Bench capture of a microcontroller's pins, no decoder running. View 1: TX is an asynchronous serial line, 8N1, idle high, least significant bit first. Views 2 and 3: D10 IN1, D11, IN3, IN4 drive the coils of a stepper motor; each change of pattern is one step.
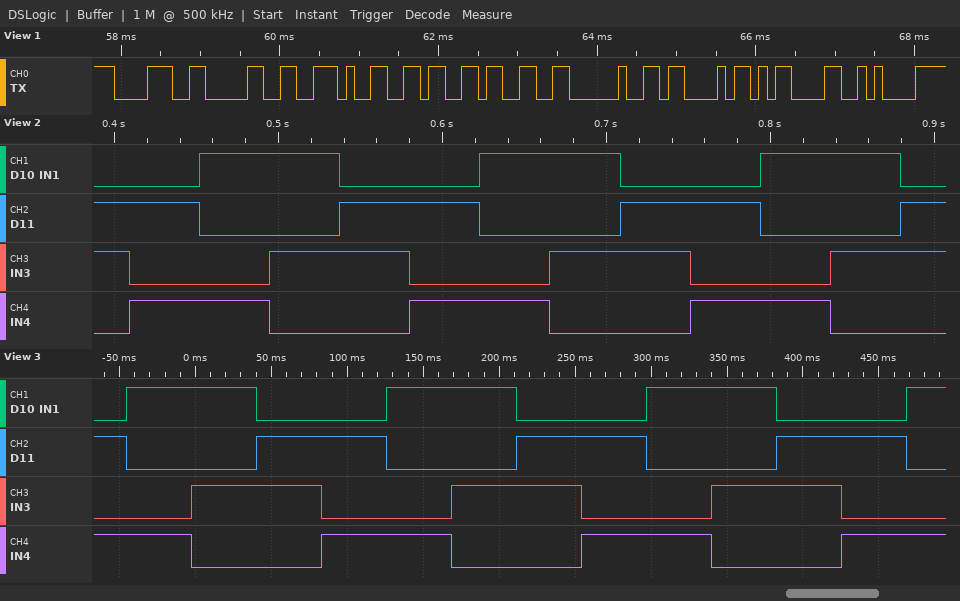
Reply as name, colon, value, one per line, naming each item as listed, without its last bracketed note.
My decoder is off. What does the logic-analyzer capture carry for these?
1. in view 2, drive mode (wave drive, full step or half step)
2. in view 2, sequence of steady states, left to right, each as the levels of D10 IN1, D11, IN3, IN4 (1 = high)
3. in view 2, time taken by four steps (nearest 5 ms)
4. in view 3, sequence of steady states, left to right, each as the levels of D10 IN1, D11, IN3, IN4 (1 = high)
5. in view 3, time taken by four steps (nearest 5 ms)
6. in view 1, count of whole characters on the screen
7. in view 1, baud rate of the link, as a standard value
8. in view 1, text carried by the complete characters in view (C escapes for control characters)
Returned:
in view 2, drive mode: full step
in view 2, sequence of steady states, left to right, each as the levels of D10 IN1, D11, IN3, IN4: 0110 0101 1001 1010 0110 0101 1001 1010 0110 0101 1001 1010 0110
in view 2, time taken by four steps: 170 ms
in view 3, sequence of steady states, left to right, each as the levels of D10 IN1, D11, IN3, IN4: 0101 1001 1010 0110 0101 1001 1010 0110 0101 1001 1010 0110 0101 1001
in view 3, time taken by four steps: 170 ms
in view 1, count of whole characters on the screen: 9
in view 1, baud rate of the link, as a standard value: 9600 baud
in view 1, text carried by the complete characters in view: "80.63 C\r\n"
